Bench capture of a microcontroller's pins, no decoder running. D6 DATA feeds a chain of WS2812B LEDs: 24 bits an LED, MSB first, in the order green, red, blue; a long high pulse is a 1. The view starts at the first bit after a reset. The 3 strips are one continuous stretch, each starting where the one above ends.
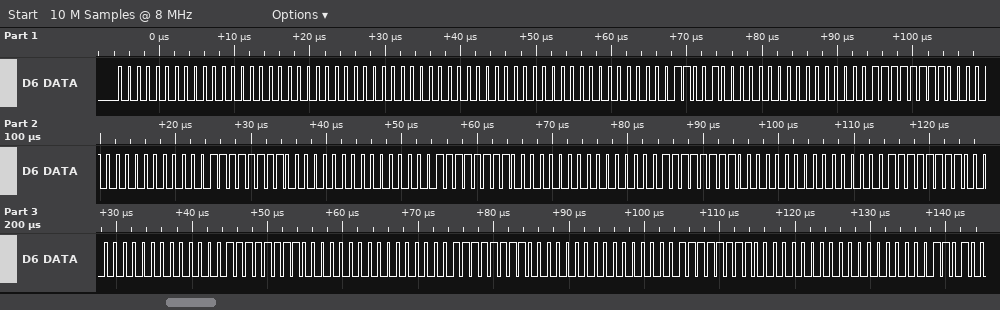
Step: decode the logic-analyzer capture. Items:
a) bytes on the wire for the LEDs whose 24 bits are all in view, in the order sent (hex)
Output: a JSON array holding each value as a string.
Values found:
["00 00 00 00 00 00 00 19 00 00 FF 00 00 FF 00 00 FF 00 00 FF 00 00 FF 00 00 FF 00 00 FF 00 00 FF 00"]
